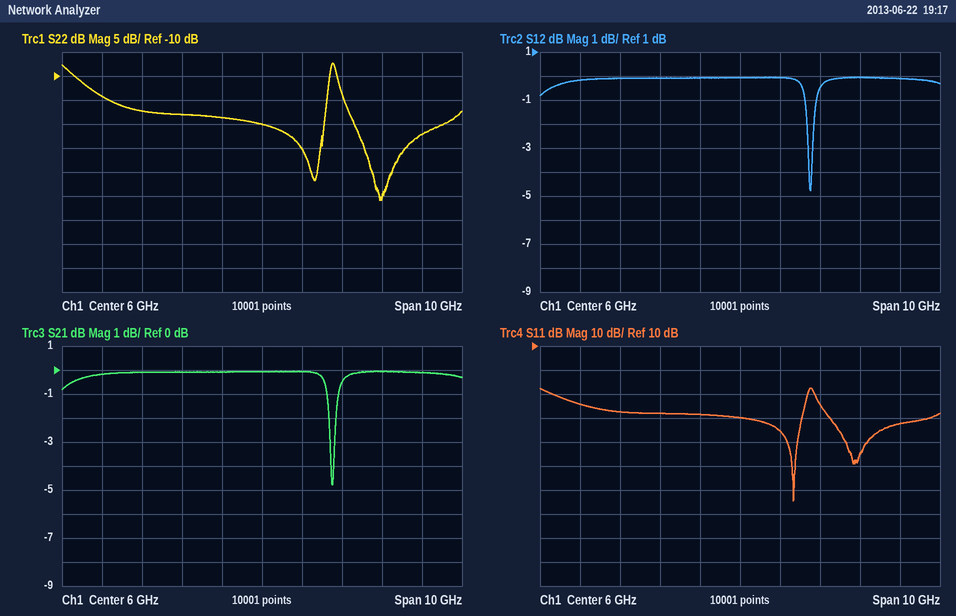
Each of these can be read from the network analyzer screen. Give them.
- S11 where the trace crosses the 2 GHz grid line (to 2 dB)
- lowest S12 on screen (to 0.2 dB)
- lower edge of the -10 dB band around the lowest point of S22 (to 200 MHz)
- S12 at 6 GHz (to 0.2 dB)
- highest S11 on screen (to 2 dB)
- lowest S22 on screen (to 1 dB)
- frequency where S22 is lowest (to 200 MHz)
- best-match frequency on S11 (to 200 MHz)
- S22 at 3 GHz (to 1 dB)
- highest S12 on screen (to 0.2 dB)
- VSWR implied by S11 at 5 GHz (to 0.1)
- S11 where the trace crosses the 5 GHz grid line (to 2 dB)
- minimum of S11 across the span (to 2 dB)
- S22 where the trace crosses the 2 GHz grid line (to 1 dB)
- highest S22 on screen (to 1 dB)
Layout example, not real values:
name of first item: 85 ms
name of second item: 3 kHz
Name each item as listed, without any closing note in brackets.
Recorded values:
S11 where the trace crosses the 2 GHz grid line: -14 dB
lowest S12 on screen: -4.8 dB
lower edge of the -10 dB band around the lowest point of S22: 7.8 GHz
S12 at 6 GHz: 0.0 dB
highest S11 on screen: -8 dB
lowest S22 on screen: -36 dB
frequency where S22 is lowest: 9.0 GHz
best-match frequency on S11: 7.4 GHz
S22 at 3 GHz: -17 dB
highest S12 on screen: 0.0 dB
VSWR implied by S11 at 5 GHz: 1.3
S11 where the trace crosses the 5 GHz grid line: -18 dB
minimum of S11 across the span: -54 dB
S22 where the trace crosses the 2 GHz grid line: -14 dB
highest S22 on screen: -7 dB
